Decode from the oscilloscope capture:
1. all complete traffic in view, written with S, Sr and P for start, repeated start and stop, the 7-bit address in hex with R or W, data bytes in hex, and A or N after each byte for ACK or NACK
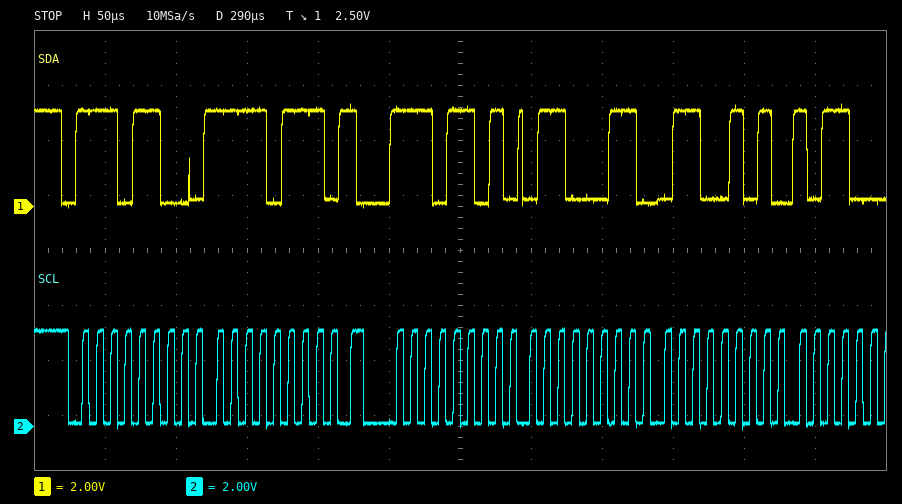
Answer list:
S 76W A F7 A Sr 76R A 63 A 65 A
